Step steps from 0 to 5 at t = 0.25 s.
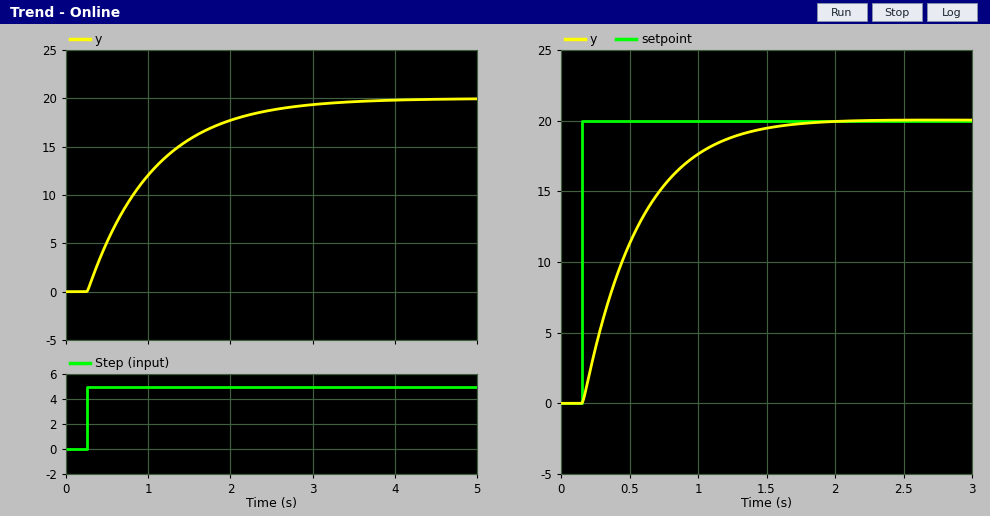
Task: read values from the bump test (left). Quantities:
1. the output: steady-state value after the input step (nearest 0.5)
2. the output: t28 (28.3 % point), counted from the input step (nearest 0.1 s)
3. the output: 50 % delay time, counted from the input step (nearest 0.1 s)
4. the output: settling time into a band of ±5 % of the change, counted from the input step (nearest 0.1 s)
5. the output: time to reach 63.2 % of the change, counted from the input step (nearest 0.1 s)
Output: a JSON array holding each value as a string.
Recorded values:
["20.0", "0.3 s", "0.6 s", "2.4 s", "0.8 s"]
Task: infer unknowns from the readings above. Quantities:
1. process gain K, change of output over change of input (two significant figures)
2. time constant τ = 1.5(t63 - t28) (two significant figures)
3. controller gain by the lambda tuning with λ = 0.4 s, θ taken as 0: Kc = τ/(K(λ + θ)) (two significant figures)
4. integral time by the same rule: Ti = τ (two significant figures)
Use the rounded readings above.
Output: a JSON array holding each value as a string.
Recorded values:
["4.0", "0.75 s", "0.47", "0.75 s"]
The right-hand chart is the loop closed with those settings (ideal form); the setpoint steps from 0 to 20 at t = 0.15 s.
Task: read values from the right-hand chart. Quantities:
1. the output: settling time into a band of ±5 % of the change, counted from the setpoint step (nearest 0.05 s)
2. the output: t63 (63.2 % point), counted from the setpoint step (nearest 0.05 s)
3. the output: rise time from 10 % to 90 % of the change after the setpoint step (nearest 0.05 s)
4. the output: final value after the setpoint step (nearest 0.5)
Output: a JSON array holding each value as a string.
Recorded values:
["1.15 s", "0.40 s", "0.85 s", "20.0"]
